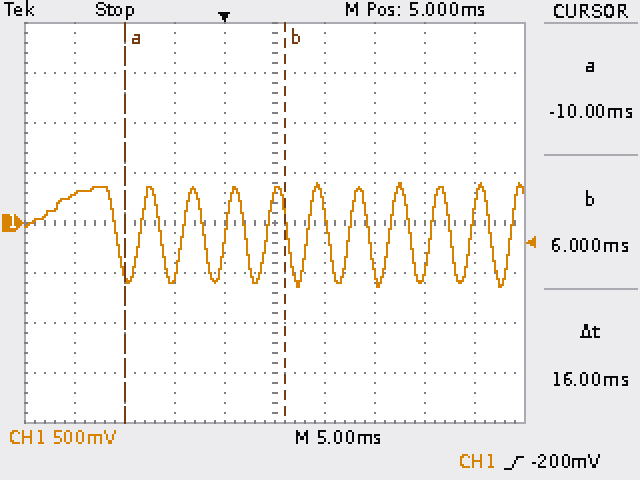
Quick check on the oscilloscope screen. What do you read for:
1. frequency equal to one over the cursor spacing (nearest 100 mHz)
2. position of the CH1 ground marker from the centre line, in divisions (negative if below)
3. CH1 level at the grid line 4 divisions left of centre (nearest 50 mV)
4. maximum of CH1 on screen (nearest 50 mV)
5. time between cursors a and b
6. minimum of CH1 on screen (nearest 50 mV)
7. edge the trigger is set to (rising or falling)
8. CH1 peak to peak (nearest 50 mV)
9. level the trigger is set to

62.5 Hz
0.0 div
300 mV
400 mV
16 ms
-650 mV
rising
1.05 V
-200 mV
